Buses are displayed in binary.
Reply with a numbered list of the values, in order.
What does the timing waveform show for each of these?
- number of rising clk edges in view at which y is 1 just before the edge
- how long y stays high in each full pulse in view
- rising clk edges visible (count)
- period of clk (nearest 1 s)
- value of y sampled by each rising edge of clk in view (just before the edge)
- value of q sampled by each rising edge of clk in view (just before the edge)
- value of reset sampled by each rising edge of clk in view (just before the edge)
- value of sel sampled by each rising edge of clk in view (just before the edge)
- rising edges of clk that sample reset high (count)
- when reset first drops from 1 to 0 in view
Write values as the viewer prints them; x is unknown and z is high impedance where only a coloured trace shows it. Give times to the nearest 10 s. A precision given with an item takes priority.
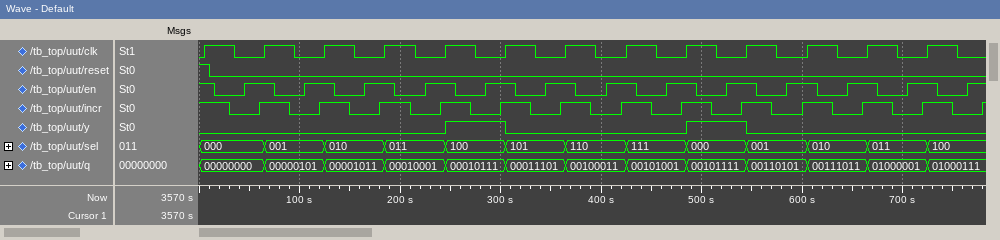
1. 2
2. 60 s, 60 s
3. 13
4. 60 s
5. 0 0 0 0 0 1 0 0 0 1 0 0 0
6. 00000000, 00000000, 00000101, 00001011, 00010001, 00010111, 00011101, 00100011, 00101001, 00101111, 00110101, 00111011, 01000001
7. 1 0 0 0 0 0 0 0 0 0 0 0 0
8. 000, 000, 001, 010, 011, 100, 101, 110, 111, 000, 001, 010, 011
9. 1
10. 10 s
